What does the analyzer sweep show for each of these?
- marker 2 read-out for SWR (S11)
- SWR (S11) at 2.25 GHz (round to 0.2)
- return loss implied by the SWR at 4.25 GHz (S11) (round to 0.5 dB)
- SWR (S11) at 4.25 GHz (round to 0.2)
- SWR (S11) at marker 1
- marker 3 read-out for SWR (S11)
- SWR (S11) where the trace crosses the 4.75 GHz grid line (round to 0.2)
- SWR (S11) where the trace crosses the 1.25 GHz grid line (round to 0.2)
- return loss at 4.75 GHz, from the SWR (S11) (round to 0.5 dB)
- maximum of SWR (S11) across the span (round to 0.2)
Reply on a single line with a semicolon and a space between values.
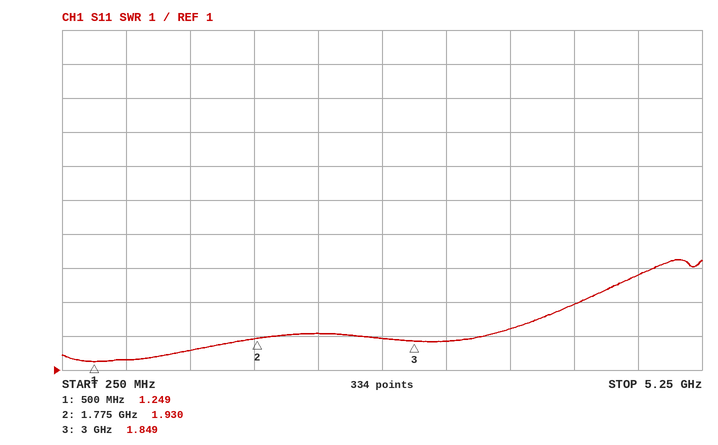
1.930; 2.0; 6.0 dB; 3.0; 1.249; 1.849; 3.8; 1.6; 4.5 dB; 4.2
